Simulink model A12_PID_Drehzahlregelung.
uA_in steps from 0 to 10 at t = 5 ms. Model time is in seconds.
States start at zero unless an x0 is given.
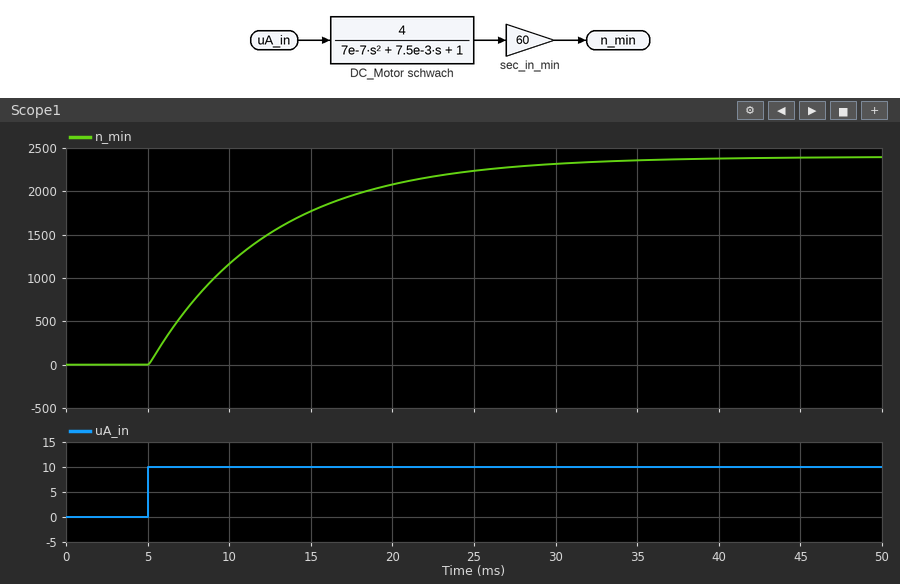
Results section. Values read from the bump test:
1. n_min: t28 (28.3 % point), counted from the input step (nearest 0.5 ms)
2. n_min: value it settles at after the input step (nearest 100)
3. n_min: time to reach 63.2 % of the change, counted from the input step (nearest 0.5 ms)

2.5 ms
2400
7.5 ms
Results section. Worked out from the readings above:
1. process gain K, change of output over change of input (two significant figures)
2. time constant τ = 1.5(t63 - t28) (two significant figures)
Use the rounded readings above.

240
7.5 ms
